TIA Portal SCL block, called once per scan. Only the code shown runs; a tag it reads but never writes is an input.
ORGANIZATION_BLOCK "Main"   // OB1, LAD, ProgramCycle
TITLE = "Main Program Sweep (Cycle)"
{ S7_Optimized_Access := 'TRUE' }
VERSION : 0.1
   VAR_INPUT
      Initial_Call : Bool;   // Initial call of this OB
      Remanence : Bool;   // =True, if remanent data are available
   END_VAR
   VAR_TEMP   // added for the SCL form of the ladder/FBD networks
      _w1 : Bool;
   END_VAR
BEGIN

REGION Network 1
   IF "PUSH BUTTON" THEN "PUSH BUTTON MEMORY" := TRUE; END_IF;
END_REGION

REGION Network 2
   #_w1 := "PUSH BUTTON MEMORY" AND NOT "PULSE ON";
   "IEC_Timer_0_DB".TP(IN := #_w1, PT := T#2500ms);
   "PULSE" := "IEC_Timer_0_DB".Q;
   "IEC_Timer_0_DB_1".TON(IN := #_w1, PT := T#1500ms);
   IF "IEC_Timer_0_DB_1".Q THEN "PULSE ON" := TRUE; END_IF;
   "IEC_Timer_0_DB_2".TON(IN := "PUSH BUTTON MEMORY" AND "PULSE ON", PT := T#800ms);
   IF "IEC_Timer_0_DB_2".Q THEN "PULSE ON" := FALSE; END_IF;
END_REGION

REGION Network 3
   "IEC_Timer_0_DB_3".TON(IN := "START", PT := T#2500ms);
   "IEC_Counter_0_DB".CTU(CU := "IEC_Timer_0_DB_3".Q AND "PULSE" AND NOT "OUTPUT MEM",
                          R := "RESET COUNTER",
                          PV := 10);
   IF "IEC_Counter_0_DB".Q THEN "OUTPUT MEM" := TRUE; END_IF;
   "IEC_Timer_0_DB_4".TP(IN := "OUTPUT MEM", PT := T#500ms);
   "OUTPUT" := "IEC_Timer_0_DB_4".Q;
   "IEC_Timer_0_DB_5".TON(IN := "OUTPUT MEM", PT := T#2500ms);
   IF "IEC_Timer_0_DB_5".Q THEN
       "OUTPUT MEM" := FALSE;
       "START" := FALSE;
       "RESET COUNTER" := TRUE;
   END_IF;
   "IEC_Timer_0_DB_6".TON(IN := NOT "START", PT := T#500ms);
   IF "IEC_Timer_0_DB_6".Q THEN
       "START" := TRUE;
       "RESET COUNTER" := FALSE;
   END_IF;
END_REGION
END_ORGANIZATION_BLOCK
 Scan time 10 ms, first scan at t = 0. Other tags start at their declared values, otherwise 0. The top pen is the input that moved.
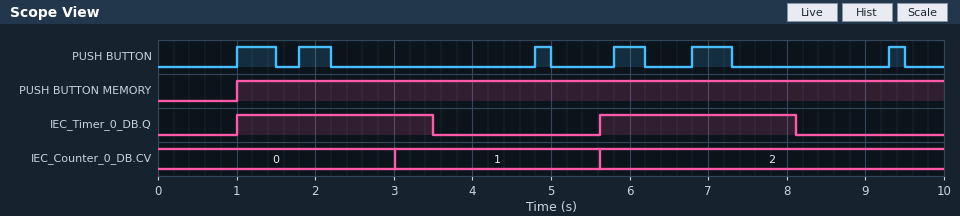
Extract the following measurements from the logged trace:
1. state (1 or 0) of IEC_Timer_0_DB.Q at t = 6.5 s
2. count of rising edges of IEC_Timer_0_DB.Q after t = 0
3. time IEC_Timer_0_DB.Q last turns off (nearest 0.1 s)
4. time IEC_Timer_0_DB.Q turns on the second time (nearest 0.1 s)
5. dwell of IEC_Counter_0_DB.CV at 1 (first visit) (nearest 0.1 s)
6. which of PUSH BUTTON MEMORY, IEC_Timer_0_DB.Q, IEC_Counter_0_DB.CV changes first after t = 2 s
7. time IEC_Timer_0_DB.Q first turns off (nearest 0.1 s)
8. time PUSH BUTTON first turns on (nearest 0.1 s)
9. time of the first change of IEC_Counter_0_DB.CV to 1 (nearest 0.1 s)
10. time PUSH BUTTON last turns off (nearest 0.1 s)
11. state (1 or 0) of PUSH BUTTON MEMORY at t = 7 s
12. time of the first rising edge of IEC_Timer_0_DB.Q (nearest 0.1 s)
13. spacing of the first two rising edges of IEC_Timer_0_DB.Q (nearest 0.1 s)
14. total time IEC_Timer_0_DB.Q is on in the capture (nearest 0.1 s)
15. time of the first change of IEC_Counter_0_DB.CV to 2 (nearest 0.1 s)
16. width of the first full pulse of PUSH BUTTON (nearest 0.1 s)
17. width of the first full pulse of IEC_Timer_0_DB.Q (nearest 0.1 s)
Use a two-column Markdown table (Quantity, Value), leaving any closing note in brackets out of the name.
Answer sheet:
| Quantity | Value |
|---|---|
| state (1 or 0) of IEC_Timer_0_DB.Q at t = 6.5 s | 1 |
| count of rising edges of IEC_Timer_0_DB.Q after t = 0 | 2 |
| time IEC_Timer_0_DB.Q last turns off | 8.1 s |
| time IEC_Timer_0_DB.Q turns on the second time | 5.6 s |
| dwell of IEC_Counter_0_DB.CV at 1 (first visit) | 2.6 s |
| which of PUSH BUTTON MEMORY, IEC_Timer_0_DB.Q, IEC_Counter_0_DB.CV changes first after t = 2 s | IEC_Counter_0_DB.CV |
| time IEC_Timer_0_DB.Q first turns off | 3.5 s |
| time PUSH BUTTON first turns on | 1.0 s |
| time of the first change of IEC_Counter_0_DB.CV to 1 | 3.0 s |
| time PUSH BUTTON last turns off | 9.5 s |
| state (1 or 0) of PUSH BUTTON MEMORY at t = 7 s | 1 |
| time of the first rising edge of IEC_Timer_0_DB.Q | 1.0 s |
| spacing of the first two rising edges of IEC_Timer_0_DB.Q | 4.6 s |
| total time IEC_Timer_0_DB.Q is on in the capture | 5.0 s |
| time of the first change of IEC_Counter_0_DB.CV to 2 | 5.6 s |
| width of the first full pulse of PUSH BUTTON | 0.5 s |
| width of the first full pulse of IEC_Timer_0_DB.Q | 2.5 s |
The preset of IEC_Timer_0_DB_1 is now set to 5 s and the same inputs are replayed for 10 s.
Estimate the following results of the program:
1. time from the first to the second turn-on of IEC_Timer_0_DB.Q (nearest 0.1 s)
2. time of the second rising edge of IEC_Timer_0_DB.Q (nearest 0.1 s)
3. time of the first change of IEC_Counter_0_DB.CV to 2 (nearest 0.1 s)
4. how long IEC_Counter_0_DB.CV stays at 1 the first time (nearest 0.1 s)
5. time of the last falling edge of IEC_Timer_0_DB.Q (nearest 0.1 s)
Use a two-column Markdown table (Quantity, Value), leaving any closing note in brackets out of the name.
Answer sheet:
| Quantity | Value |
|---|---|
| time from the first to the second turn-on of IEC_Timer_0_DB.Q | 5.8 s |
| time of the second rising edge of IEC_Timer_0_DB.Q | 6.8 s |
| time of the first change of IEC_Counter_0_DB.CV to 2 | 6.8 s |
| how long IEC_Counter_0_DB.CV stays at 1 the first time | 3.8 s |
| time of the last falling edge of IEC_Timer_0_DB.Q | 9.3 s |
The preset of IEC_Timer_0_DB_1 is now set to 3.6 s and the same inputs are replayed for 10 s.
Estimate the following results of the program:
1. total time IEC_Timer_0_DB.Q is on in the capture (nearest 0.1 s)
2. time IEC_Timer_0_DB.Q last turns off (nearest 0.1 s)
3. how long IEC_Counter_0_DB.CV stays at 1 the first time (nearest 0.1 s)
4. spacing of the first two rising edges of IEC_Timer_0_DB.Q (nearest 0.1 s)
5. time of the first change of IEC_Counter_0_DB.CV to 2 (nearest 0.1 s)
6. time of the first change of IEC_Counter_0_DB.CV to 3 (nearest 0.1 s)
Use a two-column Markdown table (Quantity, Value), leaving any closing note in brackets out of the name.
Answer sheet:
| Quantity | Value |
|---|---|
| total time IEC_Timer_0_DB.Q is on in the capture | 5.2 s |
| time IEC_Timer_0_DB.Q last turns off | 7.9 s |
| how long IEC_Counter_0_DB.CV stays at 1 the first time | 2.4 s |
| spacing of the first two rising edges of IEC_Timer_0_DB.Q | 4.4 s |
| time of the first change of IEC_Counter_0_DB.CV to 2 | 5.4 s |
| time of the first change of IEC_Counter_0_DB.CV to 3 | 9.8 s |
